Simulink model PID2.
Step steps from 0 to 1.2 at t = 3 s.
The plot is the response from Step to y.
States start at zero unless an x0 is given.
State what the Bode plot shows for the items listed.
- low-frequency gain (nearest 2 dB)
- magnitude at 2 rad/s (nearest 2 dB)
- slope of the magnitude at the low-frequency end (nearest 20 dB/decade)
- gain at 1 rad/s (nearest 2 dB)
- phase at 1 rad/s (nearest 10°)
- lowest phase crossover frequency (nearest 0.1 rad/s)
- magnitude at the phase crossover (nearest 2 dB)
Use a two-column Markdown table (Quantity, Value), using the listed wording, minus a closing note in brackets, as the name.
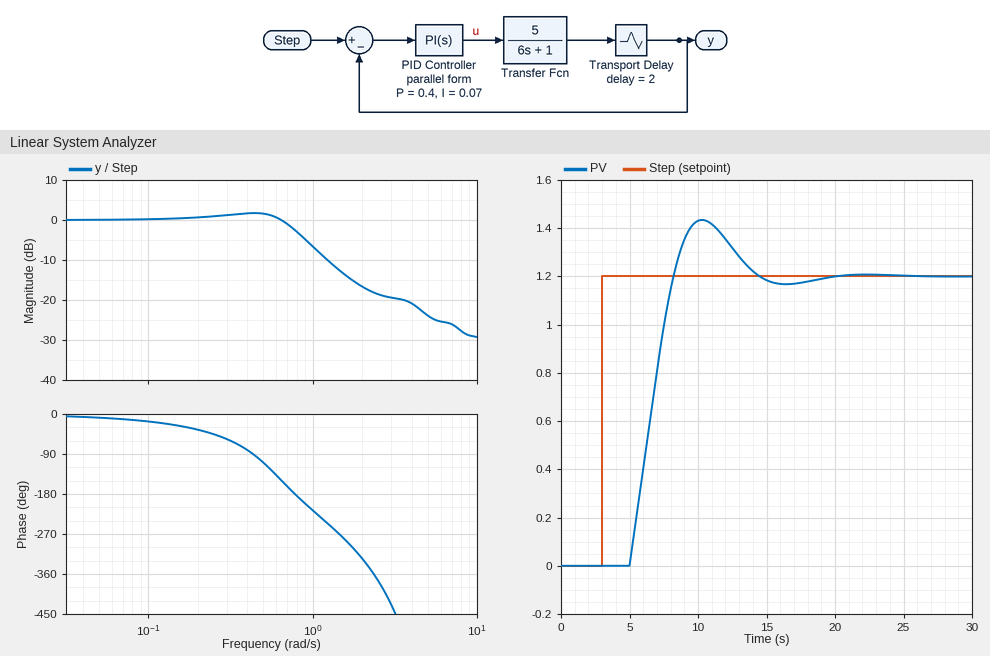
| Quantity | Value |
|---|---|
| low-frequency gain | 0 dB |
| magnitude at 2 rad/s | -16 dB |
| slope of the magnitude at the low-frequency end | 0 dB/decade |
| gain at 1 rad/s | -6 dB |
| phase at 1 rad/s | -220° |
| lowest phase crossover frequency | 0.8 rad/s |
| magnitude at the phase crossover | -2 dB |
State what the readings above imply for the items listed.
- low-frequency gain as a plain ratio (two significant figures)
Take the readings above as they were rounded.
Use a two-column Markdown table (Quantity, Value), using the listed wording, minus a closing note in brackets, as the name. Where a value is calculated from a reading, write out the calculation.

| Quantity | Value |
|---|---|
| low-frequency gain as a plain ratio | 10^(0 / 20) = 1.0 |
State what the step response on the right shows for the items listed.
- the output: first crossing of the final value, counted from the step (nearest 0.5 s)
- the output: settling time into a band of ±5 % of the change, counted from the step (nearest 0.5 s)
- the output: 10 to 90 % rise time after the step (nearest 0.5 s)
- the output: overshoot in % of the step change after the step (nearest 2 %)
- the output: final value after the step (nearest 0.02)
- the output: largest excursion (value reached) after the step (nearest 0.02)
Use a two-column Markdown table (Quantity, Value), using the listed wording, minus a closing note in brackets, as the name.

| Quantity | Value |
|---|---|
| the output: first crossing of the final value, counted from the step | 5.0 s |
| the output: settling time into a band of ±5 % of the change, counted from the step | 10.5 s |
| the output: 10 to 90 % rise time after the step | 2.5 s |
| the output: overshoot in % of the step change after the step | 20 % |
| the output: final value after the step | 1.20 |
| the output: largest excursion (value reached) after the step | 1.44 |
